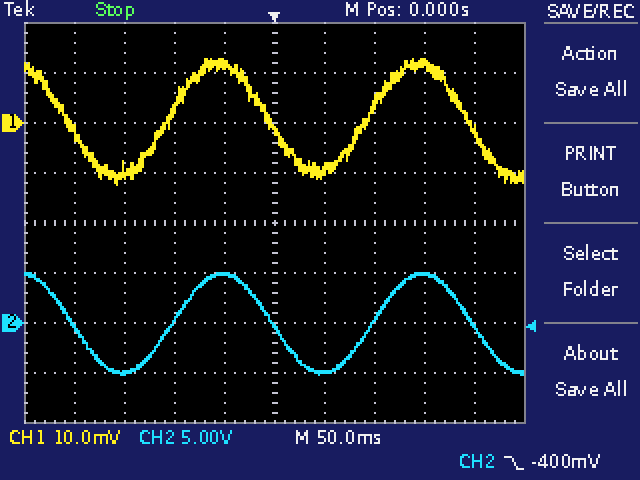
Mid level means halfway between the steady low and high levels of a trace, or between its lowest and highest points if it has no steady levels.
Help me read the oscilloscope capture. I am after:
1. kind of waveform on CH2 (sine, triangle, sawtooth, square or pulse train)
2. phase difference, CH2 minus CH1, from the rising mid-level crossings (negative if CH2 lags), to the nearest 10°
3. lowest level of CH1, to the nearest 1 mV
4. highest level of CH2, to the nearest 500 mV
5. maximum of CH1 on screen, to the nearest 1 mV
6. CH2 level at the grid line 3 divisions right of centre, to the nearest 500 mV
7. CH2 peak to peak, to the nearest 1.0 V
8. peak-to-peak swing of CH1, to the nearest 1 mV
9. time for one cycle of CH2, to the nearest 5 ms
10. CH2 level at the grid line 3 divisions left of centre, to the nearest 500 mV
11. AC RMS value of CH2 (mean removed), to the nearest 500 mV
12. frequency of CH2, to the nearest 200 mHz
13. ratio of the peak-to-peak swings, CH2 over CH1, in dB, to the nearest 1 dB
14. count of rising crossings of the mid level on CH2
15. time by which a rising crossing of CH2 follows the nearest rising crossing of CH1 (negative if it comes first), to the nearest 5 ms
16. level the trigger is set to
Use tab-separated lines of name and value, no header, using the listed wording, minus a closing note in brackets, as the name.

kind of waveform on CH2	sine
phase difference, CH2 minus CH1, from the rising mid-level crossings (negative if CH2 lags), to the nearest 10°	-10°
lowest level of CH1, to the nearest 1 mV	-12 mV
highest level of CH2, to the nearest 500 mV	5.0 V
maximum of CH1 on screen, to the nearest 1 mV	13 mV
CH2 level at the grid line 3 divisions right of centre, to the nearest 500 mV	5.0 V
CH2 peak to peak, to the nearest 1.0 V	10.0 V
peak-to-peak swing of CH1, to the nearest 1 mV	25 mV
time for one cycle of CH2, to the nearest 5 ms	200 ms
CH2 level at the grid line 3 divisions left of centre, to the nearest 500 mV	-5.0 V
AC RMS value of CH2 (mean removed), to the nearest 500 mV	3.5 V
frequency of CH2, to the nearest 200 mHz	5.0 Hz
ratio of the peak-to-peak swings, CH2 over CH1, in dB, to the nearest 1 dB	52 dB
count of rising crossings of the mid level on CH2	2
time by which a rising crossing of CH2 follows the nearest rising crossing of CH1 (negative if it comes first), to the nearest 5 ms	+5 ms
level the trigger is set to	-400 mV
